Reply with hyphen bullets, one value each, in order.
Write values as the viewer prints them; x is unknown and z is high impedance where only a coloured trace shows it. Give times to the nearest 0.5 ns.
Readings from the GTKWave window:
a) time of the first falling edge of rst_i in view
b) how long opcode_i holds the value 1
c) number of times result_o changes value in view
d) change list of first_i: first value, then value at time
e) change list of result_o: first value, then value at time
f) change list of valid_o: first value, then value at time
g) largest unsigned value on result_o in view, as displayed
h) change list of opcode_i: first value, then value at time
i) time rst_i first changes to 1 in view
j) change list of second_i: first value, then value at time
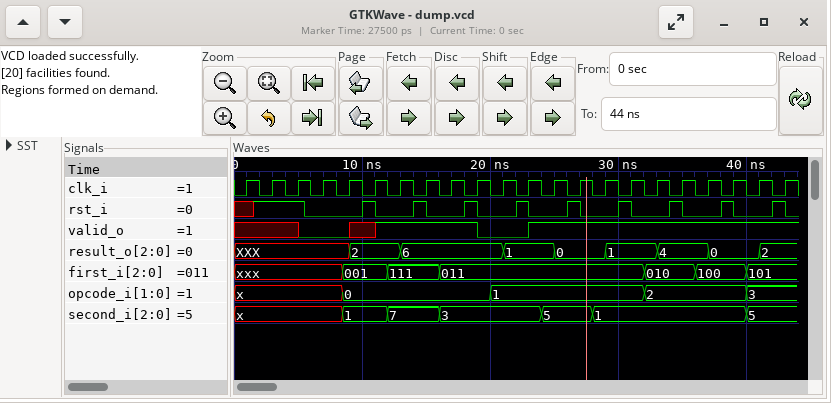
- 5.5 ns
- 12 ns
- 8
- xxx, 001 at 8.5 ns, 111 at 12 ns, 011 at 16 ns, 010 at 32 ns, 100 at 36 ns, 101 at 40 ns
- XXX, 2 at 9 ns, 6 at 13 ns, 1 at 21 ns, 0 at 25 ns, 1 at 29 ns, 4 at 33 ns, 0 at 37 ns, 2 at 41 ns
- x, 0 at 5 ns, x at 9 ns, 1 at 11 ns, 0 at 19 ns, 1 at 23 ns
- 6
- x, 0 at 8.5 ns, 1 at 20 ns, 2 at 32 ns, 3 at 40 ns
- 1.5 ns
- x, 1 at 8.5 ns, 7 at 12 ns, 3 at 16 ns, 5 at 24 ns, 1 at 28 ns, 5 at 40 ns
